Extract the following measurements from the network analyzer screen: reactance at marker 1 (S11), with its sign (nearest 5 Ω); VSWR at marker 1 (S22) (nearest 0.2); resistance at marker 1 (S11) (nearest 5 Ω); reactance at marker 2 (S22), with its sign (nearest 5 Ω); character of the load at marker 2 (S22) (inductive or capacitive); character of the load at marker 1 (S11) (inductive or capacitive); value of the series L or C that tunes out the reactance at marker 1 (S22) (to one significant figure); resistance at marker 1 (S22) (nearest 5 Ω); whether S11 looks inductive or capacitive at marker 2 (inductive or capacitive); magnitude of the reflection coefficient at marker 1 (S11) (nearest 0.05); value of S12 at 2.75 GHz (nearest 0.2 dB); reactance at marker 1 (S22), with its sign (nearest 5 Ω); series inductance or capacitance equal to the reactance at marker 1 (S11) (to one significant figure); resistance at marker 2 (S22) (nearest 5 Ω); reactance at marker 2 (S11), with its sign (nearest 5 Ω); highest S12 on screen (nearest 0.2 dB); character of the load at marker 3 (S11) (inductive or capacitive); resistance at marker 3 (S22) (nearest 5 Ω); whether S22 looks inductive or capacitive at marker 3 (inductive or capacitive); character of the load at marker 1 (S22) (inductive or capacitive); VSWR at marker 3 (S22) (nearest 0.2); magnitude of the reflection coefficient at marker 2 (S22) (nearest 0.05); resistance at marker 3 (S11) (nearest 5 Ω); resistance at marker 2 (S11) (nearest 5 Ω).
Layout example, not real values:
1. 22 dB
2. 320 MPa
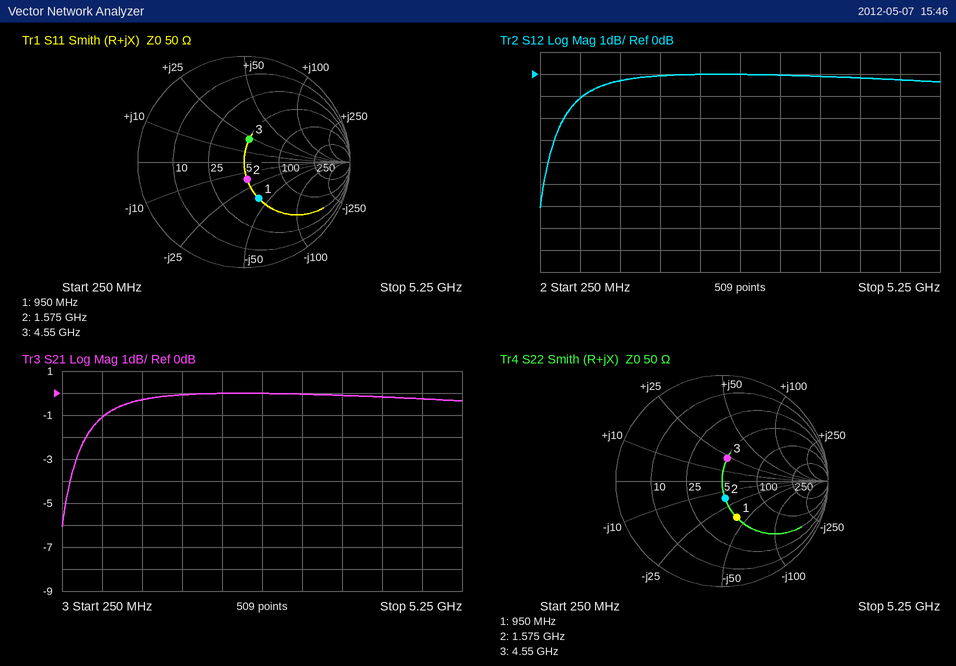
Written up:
1. -40 Ω
2. 2.2
3. 50 Ω
4. -15 Ω
5. capacitive
6. capacitive
7. 7 nH
8. 50 Ω
9. capacitive
10. 0.35
11. 0.0 dB
12. -40 Ω
13. 4 pF
14. 50 Ω
15. -15 Ω
16. 0.0 dB
17. inductive
18. 50 Ω
19. inductive
20. capacitive
21. 1.6
22. 0.15
23. 50 Ω
24. 50 Ω
